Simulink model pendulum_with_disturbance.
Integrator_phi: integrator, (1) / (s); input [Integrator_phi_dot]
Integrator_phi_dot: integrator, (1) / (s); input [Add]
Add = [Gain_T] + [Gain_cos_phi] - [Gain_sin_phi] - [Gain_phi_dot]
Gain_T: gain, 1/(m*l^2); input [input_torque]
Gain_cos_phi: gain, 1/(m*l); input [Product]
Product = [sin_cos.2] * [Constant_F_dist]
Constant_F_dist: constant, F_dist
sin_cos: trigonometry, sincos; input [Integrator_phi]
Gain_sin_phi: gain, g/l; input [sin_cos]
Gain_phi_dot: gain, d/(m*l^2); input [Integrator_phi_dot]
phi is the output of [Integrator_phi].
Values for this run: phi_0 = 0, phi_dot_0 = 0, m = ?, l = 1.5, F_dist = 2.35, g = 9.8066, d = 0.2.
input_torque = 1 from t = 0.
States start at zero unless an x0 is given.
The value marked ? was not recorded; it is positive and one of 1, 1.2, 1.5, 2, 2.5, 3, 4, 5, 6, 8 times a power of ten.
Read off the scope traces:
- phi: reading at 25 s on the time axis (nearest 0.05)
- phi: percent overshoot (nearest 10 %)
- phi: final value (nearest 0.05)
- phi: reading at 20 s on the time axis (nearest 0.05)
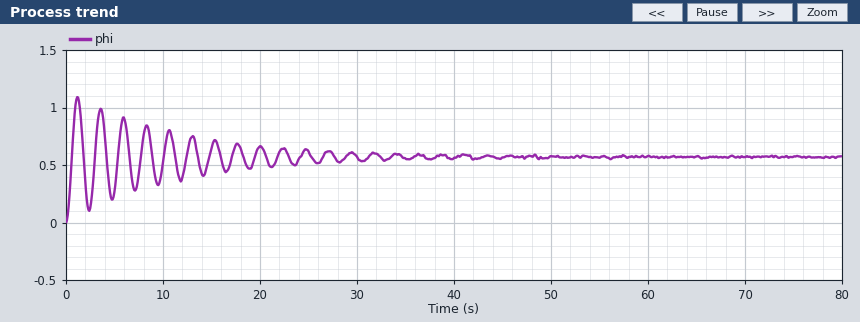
0.60
90 %
0.55
0.65
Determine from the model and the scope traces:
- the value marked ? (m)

0.5
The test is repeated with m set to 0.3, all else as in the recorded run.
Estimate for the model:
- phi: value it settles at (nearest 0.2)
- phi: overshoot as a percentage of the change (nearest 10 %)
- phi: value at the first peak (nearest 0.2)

0.8
90 %
1.6
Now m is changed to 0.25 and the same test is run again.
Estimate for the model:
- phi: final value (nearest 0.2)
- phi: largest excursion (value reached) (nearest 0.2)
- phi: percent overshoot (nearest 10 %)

1.0
1.8
90 %
